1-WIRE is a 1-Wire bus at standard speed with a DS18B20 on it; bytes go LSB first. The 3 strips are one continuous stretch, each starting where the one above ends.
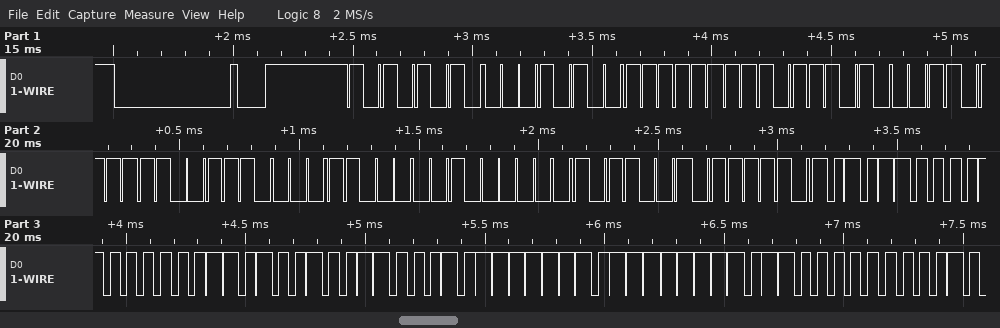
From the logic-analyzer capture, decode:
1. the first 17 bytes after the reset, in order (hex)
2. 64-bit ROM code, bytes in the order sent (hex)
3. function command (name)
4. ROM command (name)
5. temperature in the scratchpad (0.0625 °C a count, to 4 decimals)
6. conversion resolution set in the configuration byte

55 28 FF 5D EC 73 18 04 9A BE 1A 02 4B 46 7F FF 06
28 FF 5D EC 73 18 04 9A
Read Scratchpad
Match ROM
33.6250 °C
12 bits
